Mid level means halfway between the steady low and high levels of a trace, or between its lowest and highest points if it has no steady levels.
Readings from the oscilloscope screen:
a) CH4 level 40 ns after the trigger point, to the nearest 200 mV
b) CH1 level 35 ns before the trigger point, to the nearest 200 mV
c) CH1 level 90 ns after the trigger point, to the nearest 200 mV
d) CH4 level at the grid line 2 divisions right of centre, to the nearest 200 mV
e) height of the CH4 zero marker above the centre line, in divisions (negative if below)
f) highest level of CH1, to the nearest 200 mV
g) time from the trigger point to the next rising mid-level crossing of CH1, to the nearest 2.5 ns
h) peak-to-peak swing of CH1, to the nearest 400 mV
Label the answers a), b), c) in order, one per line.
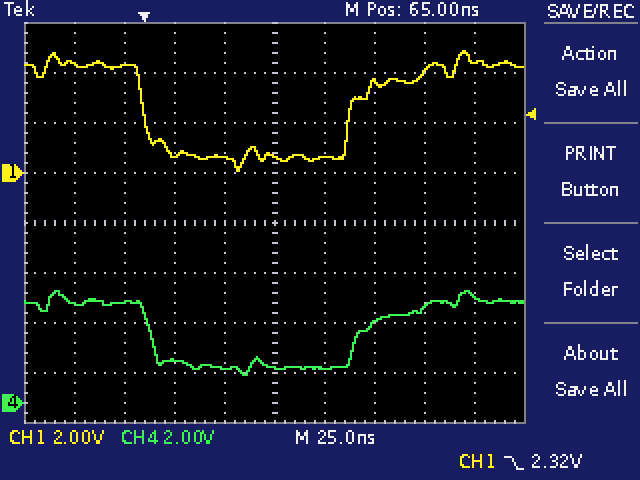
a) 1.4 V
b) 4.4 V
c) 600 mV
d) 3.2 V
e) -3.6 div
f) 4.8 V
g) 102.5 ns
h) 4.8 V
